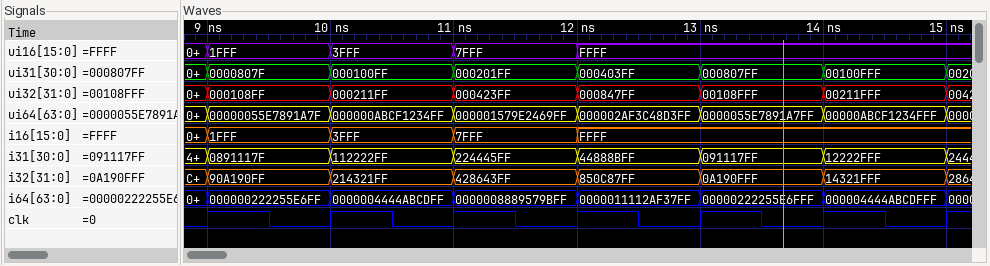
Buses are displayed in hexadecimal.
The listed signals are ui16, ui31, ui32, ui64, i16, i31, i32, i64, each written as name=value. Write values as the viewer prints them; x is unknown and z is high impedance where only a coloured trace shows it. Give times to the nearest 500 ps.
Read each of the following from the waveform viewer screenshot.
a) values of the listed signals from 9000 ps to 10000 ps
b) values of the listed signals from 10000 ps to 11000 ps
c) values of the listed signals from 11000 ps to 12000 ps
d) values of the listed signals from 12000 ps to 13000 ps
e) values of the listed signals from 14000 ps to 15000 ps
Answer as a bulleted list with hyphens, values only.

- ui16=1FFF, ui31=0000807F, ui32=000108FF, ui64=00000055E7891A7F, i16=1FFF, i31=0891117F, i32=90A190FF, i64=000000222255E6FF
- ui16=3FFF, ui31=000100FF, ui32=000211FF, ui64=000000ABCF1234FF, i16=3FFF, i31=112222FF, i32=214321FF, i64=0000004444ABCDFF
- ui16=7FFF, ui31=000201FF, ui32=000423FF, ui64=000001579E2469FF, i16=7FFF, i31=224445FF, i32=428643FF, i64=0000008889579BFF
- ui16=FFFF, ui31=000403FF, ui32=000847FF, ui64=000002AF3C48D3FF, i16=FFFF, i31=44888BFF, i32=850C87FF, i64=0000011112AF37FF
- ui16=FFFF, ui31=00100FFF, ui32=00211FFF, ui64=00000ABCF1234FFF, i16=FFFF, i31=12222FFF, i32=14321FFF, i64=000004444ABCDFFF
